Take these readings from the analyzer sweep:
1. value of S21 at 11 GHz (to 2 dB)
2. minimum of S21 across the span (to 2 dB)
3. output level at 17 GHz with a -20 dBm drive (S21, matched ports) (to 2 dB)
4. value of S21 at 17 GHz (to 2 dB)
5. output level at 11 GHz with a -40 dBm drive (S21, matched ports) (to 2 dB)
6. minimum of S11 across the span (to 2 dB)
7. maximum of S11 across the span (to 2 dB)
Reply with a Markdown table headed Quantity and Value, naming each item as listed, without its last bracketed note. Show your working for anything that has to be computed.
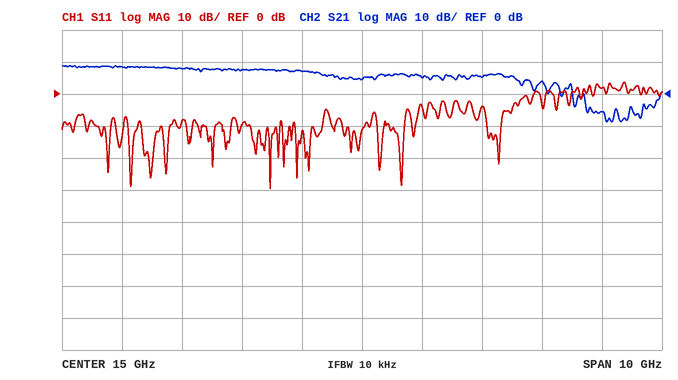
| Quantity | Value |
|---|---|
| value of S21 at 11 GHz | 8 dB |
| minimum of S21 across the span | -8 dB |
| output level at 17 GHz with a -20 dBm drive (S21, matched ports) | -20 dBm + (6 dB) = -14 dBm |
| value of S21 at 17 GHz | 6 dB |
| output level at 11 GHz with a -40 dBm drive (S21, matched ports) | -40 dBm + (8 dB) = -32 dBm |
| minimum of S11 across the span | -30 dB |
| maximum of S11 across the span | 4 dB |
